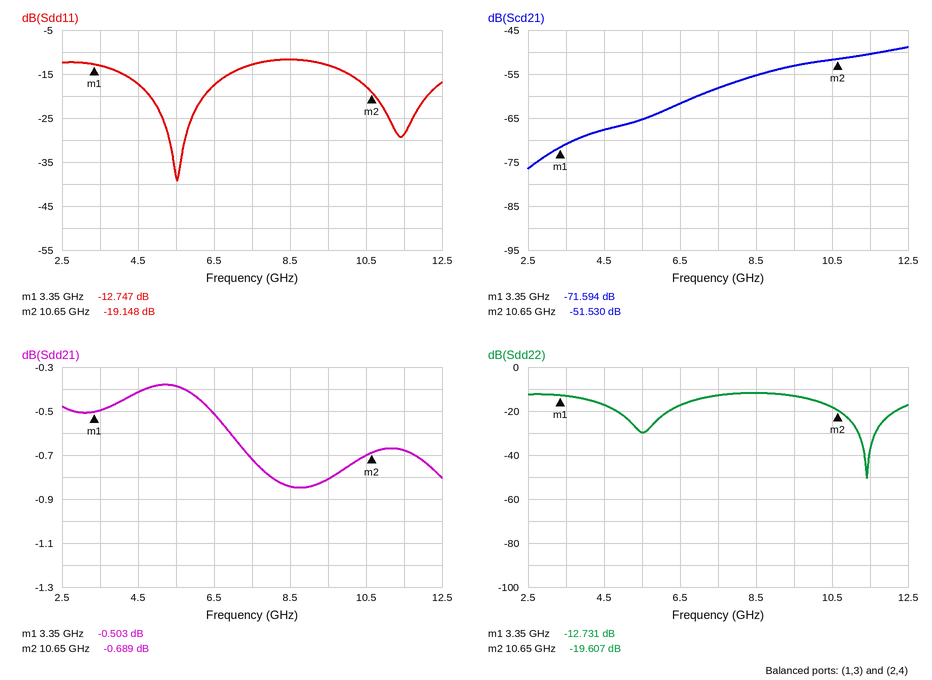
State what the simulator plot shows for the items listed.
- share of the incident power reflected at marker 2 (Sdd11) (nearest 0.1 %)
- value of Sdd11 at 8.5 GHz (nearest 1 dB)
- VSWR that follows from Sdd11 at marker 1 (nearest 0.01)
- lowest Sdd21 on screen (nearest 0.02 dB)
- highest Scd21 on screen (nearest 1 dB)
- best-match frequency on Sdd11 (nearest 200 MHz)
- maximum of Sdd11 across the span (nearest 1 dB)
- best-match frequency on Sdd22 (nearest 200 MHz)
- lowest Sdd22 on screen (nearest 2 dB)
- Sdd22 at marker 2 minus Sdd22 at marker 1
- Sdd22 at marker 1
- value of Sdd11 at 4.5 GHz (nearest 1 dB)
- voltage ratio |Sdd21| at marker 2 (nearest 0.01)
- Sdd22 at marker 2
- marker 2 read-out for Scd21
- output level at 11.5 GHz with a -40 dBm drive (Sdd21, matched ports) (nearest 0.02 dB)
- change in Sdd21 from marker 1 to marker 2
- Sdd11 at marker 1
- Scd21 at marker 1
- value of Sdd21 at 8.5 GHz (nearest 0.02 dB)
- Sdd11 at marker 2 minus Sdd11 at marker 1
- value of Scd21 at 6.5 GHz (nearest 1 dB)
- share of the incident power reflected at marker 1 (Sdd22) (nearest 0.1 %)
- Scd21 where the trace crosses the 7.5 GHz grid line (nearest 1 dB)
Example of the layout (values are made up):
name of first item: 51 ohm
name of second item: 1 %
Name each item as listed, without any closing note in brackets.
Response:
share of the incident power reflected at marker 2 (Sdd11): 1.2 %
value of Sdd11 at 8.5 GHz: -12 dB
VSWR that follows from Sdd11 at marker 1: 1.60
lowest Sdd21 on screen: -0.84 dB
highest Scd21 on screen: -49 dB
best-match frequency on Sdd11: 5.6 GHz
maximum of Sdd11 across the span: -12 dB
best-match frequency on Sdd22: 11.4 GHz
lowest Sdd22 on screen: -50 dB
Sdd22 at marker 2 minus Sdd22 at marker 1: -6.876 dB
Sdd22 at marker 1: -12.731 dB
value of Sdd11 at 4.5 GHz: -17 dB
voltage ratio |Sdd21| at marker 2: 0.92
Sdd22 at marker 2: -19.607 dB
marker 2 read-out for Scd21: -51.530 dB
output level at 11.5 GHz with a -40 dBm drive (Sdd21, matched ports): -40.68 dBm
change in Sdd21 from marker 1 to marker 2: -0.186 dB
Sdd11 at marker 1: -12.747 dB
Scd21 at marker 1: -71.594 dB
value of Sdd21 at 8.5 GHz: -0.84 dB
Sdd11 at marker 2 minus Sdd11 at marker 1: -6.401 dB
value of Scd21 at 6.5 GHz: -62 dB
share of the incident power reflected at marker 1 (Sdd22): 5.3 %
Scd21 where the trace crosses the 7.5 GHz grid line: -58 dB
